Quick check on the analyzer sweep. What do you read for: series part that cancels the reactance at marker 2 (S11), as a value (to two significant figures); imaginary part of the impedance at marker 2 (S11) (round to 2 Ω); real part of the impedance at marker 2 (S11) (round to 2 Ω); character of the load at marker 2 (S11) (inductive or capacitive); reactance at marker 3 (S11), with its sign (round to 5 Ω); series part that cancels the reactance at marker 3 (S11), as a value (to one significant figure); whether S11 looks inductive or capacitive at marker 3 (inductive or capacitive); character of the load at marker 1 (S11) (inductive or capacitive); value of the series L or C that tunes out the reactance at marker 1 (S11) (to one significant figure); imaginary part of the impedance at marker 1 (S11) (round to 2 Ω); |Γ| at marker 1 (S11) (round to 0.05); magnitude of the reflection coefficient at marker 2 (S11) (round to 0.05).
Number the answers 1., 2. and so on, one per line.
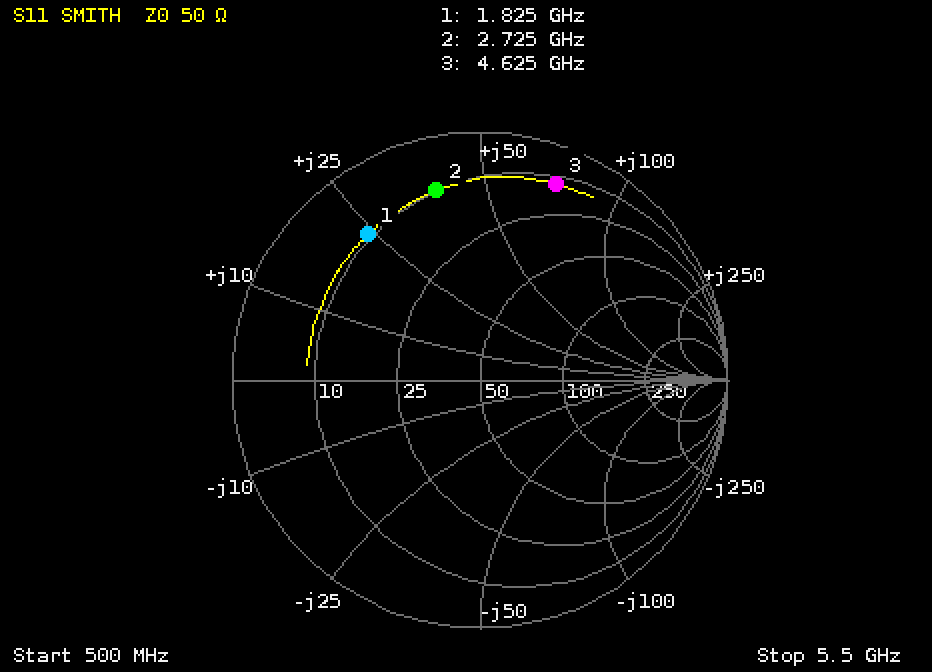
1. 1.5 pF
2. +38 Ω
3. 10 Ω
4. inductive
5. +70 Ω
6. 500 fF
7. inductive
8. inductive
9. 4 pF
10. +24 Ω
11. 0.75
12. 0.80
